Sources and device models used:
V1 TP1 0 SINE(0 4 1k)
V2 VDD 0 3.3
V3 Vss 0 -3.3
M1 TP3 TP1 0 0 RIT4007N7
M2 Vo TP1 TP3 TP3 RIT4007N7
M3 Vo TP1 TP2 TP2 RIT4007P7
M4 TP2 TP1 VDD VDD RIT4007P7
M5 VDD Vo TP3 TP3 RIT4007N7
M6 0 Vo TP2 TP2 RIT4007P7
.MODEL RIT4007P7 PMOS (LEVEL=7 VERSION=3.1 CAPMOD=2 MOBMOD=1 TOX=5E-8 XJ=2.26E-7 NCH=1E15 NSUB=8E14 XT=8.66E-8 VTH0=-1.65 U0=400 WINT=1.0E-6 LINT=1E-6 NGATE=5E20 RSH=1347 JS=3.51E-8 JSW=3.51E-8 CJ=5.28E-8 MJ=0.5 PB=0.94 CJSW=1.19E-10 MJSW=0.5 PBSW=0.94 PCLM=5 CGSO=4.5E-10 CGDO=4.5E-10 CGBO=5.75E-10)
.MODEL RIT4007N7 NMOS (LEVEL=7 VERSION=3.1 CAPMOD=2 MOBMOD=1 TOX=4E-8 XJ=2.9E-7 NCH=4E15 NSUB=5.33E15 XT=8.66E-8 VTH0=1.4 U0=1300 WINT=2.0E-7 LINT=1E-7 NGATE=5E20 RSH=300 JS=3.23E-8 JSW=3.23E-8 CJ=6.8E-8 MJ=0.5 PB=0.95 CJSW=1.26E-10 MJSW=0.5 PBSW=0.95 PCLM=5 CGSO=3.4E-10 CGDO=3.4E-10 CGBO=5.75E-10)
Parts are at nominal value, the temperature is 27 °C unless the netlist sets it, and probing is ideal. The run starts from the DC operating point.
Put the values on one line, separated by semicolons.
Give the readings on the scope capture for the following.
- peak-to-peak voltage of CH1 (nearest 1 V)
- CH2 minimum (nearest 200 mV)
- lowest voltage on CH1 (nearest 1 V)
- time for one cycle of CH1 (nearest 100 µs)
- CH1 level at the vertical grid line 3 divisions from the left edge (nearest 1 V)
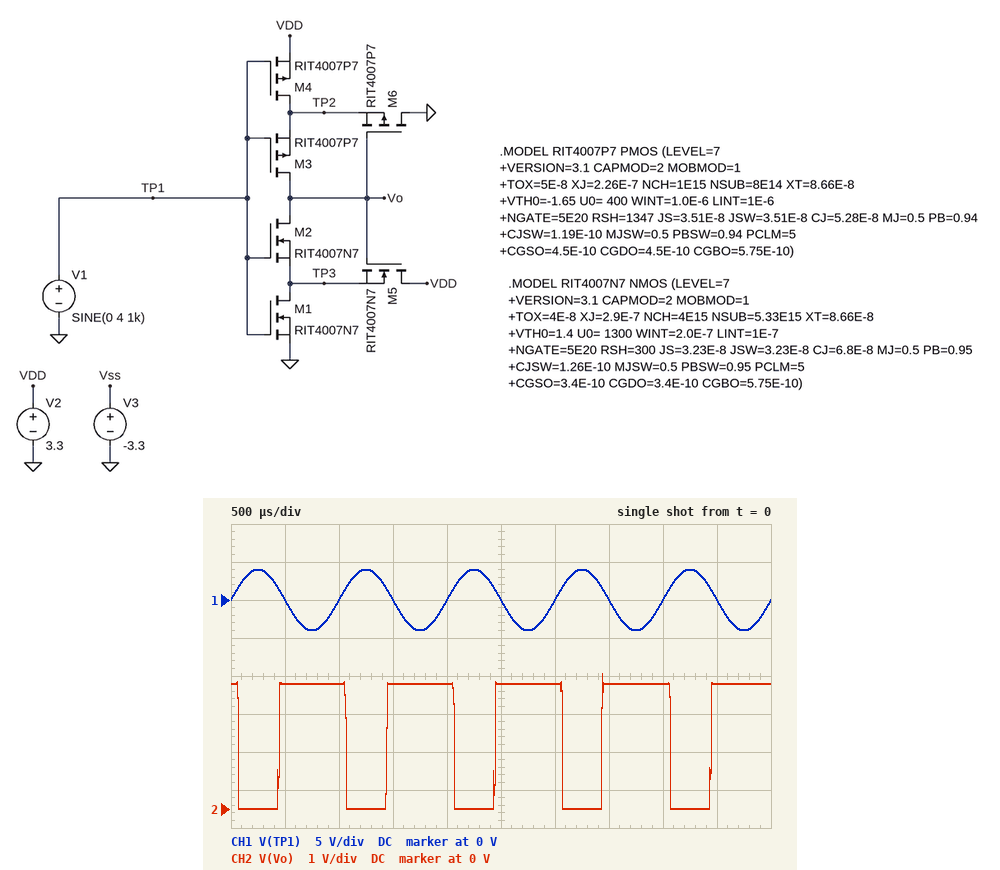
8 V; 0 V; -4 V; 1.0 ms; 0 V
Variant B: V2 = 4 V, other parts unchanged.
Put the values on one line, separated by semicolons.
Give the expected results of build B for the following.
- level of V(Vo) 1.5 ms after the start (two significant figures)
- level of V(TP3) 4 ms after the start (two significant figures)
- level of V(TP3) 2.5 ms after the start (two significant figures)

4.0 V; 4.3 V; 2.5 V
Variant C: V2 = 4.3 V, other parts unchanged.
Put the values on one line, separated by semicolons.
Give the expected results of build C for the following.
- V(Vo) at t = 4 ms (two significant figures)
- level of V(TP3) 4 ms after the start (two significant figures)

4.3 V; 4.6 V
